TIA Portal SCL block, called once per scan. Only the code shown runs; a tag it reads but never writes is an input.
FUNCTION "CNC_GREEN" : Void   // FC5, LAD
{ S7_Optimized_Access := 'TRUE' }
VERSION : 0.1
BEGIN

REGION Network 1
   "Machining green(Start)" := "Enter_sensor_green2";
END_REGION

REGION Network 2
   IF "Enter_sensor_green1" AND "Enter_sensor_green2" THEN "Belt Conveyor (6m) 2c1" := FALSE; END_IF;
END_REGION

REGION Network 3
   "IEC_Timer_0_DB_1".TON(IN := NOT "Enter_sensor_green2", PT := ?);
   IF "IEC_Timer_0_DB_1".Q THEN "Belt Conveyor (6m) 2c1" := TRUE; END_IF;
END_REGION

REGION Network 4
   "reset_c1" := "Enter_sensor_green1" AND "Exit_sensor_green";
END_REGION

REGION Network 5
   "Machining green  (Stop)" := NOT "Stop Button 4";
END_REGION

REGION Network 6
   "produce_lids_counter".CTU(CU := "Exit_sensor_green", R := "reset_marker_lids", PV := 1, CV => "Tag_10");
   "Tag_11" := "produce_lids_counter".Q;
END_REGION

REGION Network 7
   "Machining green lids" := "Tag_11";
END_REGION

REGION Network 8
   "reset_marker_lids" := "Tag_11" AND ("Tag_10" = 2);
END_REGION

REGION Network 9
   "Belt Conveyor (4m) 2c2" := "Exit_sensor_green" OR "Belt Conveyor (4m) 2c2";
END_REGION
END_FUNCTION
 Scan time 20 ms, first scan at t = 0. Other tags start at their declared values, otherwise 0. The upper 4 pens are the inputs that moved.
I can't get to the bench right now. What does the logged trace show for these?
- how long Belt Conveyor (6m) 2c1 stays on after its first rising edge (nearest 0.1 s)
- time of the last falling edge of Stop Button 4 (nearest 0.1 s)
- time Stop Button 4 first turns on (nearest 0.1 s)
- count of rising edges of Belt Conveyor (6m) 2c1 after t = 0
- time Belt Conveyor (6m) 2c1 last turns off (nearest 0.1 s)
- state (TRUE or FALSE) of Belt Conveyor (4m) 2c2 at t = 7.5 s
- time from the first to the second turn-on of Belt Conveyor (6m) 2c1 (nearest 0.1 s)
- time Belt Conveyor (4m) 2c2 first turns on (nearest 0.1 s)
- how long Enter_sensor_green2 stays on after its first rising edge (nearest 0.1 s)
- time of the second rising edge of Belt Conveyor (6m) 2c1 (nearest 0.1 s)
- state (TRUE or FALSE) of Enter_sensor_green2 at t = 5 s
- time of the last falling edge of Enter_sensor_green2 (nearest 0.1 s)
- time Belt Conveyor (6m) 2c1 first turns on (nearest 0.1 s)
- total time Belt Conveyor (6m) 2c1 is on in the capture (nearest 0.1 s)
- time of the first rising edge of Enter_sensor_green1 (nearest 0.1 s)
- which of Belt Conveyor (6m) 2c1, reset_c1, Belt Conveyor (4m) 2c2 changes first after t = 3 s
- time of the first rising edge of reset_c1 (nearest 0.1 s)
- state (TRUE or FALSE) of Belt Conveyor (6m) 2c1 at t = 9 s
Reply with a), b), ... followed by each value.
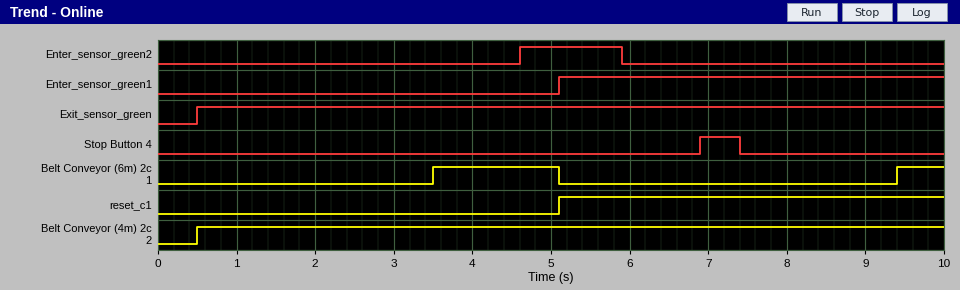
a) 1.6 s
b) 7.4 s
c) 6.9 s
d) 2
e) 5.1 s
f) TRUE
g) 5.9 s
h) 0.5 s
i) 1.3 s
j) 9.4 s
k) TRUE
l) 5.9 s
m) 3.5 s
n) 2.2 s
o) 5.1 s
p) Belt Conveyor (6m) 2c1
q) 5.1 s
r) FALSE
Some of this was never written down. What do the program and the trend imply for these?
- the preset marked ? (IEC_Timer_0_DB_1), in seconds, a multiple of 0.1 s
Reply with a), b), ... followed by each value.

a) 3.5 s
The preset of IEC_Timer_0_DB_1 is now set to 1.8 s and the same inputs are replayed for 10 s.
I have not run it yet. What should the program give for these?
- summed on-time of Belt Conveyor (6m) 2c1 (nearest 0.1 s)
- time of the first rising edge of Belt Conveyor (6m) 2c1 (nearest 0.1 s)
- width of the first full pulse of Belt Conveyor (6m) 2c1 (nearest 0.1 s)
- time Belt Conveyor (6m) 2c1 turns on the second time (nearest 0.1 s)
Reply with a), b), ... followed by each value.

a) 5.6 s
b) 1.8 s
c) 3.3 s
d) 7.7 s
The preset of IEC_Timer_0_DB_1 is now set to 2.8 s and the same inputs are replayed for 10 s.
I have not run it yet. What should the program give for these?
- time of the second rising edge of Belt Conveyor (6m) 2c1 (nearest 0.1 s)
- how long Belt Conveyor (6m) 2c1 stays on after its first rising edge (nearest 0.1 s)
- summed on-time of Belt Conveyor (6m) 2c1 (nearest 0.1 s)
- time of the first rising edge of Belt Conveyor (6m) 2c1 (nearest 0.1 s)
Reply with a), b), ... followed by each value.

a) 8.7 s
b) 2.3 s
c) 3.6 s
d) 2.8 s
